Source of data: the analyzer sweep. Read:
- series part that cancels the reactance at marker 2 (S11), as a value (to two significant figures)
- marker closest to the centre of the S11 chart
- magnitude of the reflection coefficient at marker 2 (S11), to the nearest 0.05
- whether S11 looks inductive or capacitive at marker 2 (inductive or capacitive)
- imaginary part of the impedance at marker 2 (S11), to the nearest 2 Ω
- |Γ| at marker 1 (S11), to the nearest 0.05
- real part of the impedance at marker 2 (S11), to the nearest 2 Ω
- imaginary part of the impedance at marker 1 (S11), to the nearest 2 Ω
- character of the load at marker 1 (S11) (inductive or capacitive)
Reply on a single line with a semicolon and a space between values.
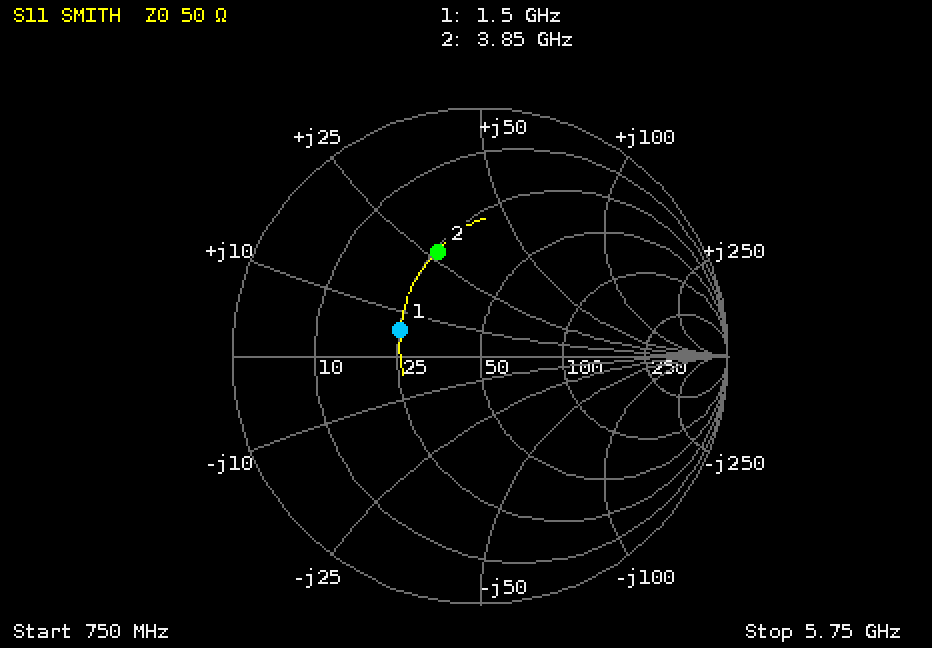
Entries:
1.5 pF; marker 1; 0.45; inductive; +28 Ω; 0.35; 26 Ω; +6 Ω; inductive
